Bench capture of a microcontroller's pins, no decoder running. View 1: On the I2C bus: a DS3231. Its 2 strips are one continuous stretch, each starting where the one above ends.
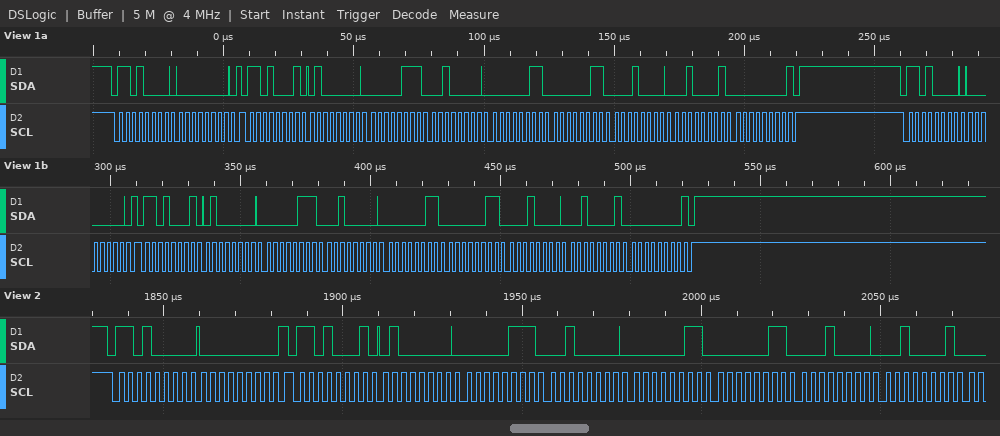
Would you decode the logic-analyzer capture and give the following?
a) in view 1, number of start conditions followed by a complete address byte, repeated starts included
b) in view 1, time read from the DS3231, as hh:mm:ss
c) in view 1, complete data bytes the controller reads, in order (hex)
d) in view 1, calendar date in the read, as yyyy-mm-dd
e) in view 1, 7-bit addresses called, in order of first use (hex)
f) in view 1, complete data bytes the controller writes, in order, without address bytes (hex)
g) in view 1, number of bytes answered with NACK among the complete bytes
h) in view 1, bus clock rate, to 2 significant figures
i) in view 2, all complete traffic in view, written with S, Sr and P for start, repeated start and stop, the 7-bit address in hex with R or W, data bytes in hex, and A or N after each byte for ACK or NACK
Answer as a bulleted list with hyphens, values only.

- 4
- 20:07:40
- 40 07 20 03 03 10 21 00 40 07 20 03 03 10 21 00
- 2021-10-03
- 0x68
- 00 00
- 2
- 400 kHz
- S 68W A 00 A Sr 68R A 40 A 07 A 20 A 03 A 03 A 10 A 21 A
